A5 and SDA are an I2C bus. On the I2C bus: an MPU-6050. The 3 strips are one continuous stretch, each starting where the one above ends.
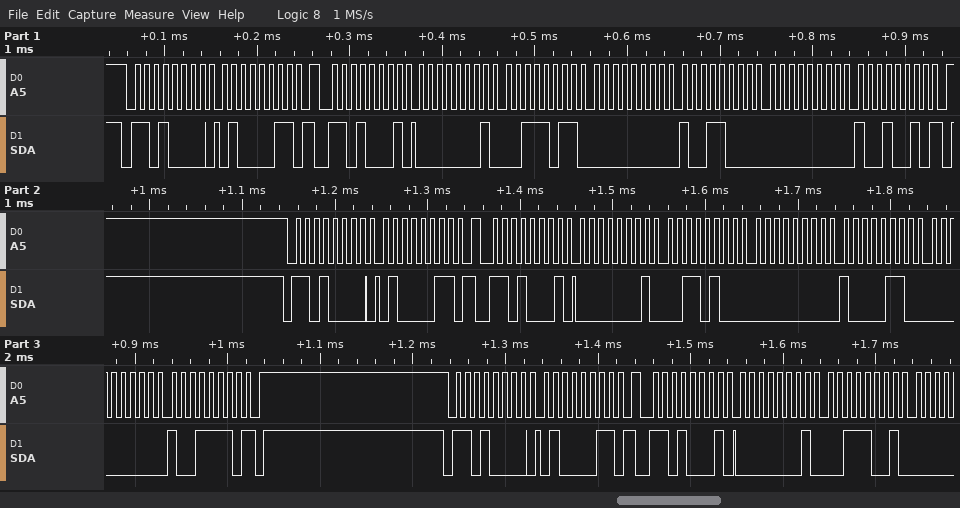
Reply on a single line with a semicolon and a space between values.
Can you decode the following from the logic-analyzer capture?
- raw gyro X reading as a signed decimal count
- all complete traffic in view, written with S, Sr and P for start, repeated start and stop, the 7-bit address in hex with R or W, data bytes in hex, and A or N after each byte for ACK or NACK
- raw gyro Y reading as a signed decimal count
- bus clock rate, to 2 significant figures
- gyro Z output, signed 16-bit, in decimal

315; S 68W A 43 A Sr 68R A 01 A 3B A 00 A 98 A 00 A 92 N P S 68W A 43 A Sr 68R A 01 A 34 A 00 A 86 A 00 A 9E N P S 68W A 43 A Sr 68R A 01 A 39 A; 152; 100 kHz; 146
